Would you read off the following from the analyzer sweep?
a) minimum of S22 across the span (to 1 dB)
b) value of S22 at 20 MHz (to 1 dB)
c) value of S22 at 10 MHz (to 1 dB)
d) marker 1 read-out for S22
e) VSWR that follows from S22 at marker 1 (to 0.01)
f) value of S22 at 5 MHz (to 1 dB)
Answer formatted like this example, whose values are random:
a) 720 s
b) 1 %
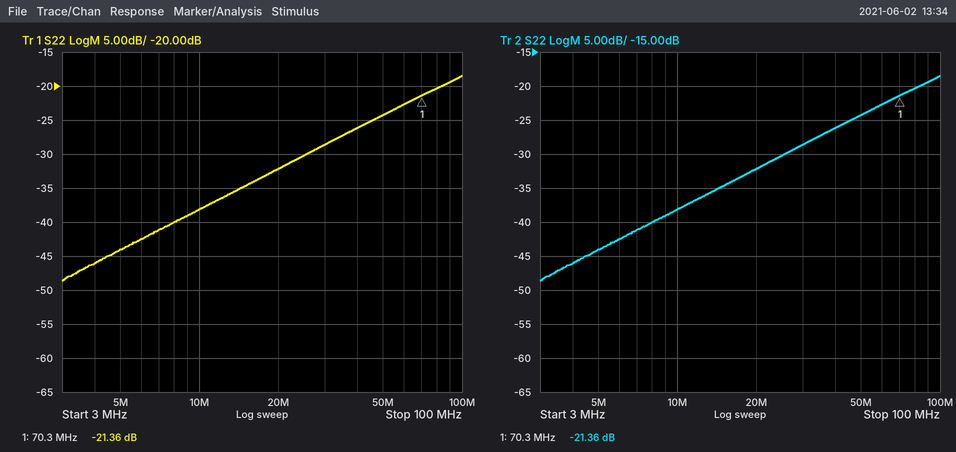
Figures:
a) -49 dB
b) -32 dB
c) -38 dB
d) -21.36 dB
e) 1.19
f) -44 dB
